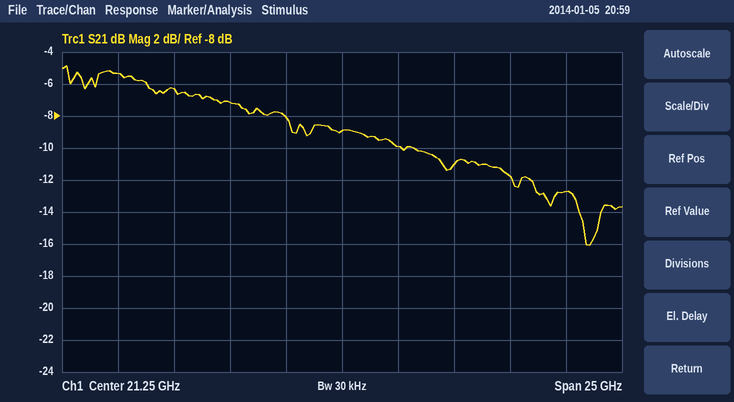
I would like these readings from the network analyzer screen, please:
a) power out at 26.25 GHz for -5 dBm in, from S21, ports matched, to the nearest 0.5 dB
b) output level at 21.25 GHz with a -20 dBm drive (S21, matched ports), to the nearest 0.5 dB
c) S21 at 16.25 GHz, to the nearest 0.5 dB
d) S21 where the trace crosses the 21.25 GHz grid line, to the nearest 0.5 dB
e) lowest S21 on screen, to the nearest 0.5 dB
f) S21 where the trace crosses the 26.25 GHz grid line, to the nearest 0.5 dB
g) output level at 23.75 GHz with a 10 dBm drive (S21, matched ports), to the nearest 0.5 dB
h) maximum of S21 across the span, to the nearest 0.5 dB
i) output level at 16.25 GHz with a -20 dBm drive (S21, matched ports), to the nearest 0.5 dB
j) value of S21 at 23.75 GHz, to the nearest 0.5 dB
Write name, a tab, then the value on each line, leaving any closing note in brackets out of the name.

power out at 26.25 GHz for -5 dBm in, from S21, ports matched, to the nearest 0.5 dB	-16.0 dBm
output level at 21.25 GHz with a -20 dBm drive (S21, matched ports), to the nearest 0.5 dB	-29.0 dBm
S21 at 16.25 GHz, to the nearest 0.5 dB	-7.0 dB
S21 where the trace crosses the 21.25 GHz grid line, to the nearest 0.5 dB	-9.0 dB
lowest S21 on screen, to the nearest 0.5 dB	-16.0 dB
S21 where the trace crosses the 26.25 GHz grid line, to the nearest 0.5 dB	-11.0 dB
output level at 23.75 GHz with a 10 dBm drive (S21, matched ports), to the nearest 0.5 dB	0.0 dBm
maximum of S21 across the span, to the nearest 0.5 dB	-5.0 dB
output level at 16.25 GHz with a -20 dBm drive (S21, matched ports), to the nearest 0.5 dB	-27.0 dBm
value of S21 at 23.75 GHz, to the nearest 0.5 dB	-10.0 dB
